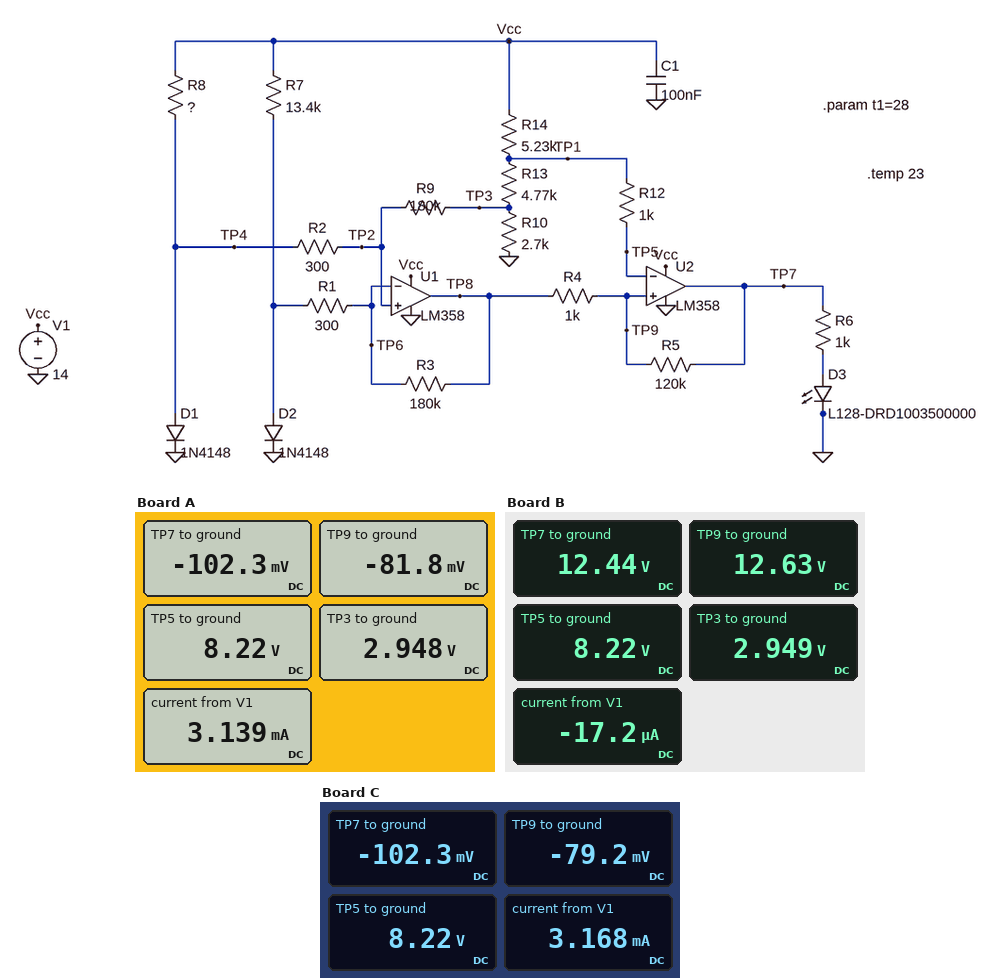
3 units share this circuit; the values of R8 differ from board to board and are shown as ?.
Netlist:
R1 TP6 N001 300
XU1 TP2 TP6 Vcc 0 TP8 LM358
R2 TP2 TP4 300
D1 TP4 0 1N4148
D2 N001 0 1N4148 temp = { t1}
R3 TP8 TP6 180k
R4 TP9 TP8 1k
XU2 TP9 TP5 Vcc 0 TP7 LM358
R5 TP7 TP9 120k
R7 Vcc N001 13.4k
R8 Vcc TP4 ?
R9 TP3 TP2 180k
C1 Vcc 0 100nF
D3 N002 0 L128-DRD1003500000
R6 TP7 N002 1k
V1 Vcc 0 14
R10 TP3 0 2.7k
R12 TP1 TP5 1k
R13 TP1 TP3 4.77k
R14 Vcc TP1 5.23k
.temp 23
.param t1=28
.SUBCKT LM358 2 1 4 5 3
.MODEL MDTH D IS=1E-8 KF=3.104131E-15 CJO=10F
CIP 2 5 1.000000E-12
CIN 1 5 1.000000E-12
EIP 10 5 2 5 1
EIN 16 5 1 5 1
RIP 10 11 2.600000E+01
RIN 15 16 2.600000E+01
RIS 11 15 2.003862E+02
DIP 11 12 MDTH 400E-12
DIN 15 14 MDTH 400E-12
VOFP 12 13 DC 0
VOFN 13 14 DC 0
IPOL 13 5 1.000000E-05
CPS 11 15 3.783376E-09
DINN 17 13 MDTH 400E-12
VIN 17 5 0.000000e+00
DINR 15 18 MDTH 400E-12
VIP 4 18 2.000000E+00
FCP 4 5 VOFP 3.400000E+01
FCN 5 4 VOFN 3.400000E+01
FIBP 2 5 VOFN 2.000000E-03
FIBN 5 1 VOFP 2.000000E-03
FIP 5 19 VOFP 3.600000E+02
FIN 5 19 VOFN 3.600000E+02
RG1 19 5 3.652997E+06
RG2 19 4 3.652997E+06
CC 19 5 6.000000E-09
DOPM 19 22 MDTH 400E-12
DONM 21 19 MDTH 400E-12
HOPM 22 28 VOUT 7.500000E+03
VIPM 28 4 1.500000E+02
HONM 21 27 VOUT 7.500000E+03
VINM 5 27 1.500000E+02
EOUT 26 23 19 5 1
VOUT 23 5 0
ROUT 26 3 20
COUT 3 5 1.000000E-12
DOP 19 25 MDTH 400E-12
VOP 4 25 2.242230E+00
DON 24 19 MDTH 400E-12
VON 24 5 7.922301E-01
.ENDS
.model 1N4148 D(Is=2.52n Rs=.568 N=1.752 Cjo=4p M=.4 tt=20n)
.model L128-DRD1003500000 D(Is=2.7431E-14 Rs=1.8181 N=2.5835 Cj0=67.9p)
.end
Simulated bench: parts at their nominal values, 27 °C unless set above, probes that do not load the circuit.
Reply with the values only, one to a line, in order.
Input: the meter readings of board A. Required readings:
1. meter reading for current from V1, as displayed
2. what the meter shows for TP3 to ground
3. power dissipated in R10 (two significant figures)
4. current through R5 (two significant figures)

3.139 mA
2.948 V
3.2 mW
170 nA
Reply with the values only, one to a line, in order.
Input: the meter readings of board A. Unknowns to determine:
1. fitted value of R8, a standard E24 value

39 kΩ
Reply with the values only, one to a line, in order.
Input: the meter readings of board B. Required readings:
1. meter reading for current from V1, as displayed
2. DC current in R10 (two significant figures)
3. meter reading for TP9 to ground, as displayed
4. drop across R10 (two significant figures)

-17.2 µA
1.1 mA
12.63 V
2.9 V
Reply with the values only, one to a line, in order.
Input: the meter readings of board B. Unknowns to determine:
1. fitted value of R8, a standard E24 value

5.6 kΩ
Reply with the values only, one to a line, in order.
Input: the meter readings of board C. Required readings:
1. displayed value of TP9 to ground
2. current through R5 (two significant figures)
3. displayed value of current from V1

-79.2 mV
190 nA
3.168 mA
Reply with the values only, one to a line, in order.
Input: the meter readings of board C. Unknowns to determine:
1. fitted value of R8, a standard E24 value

36 kΩ
